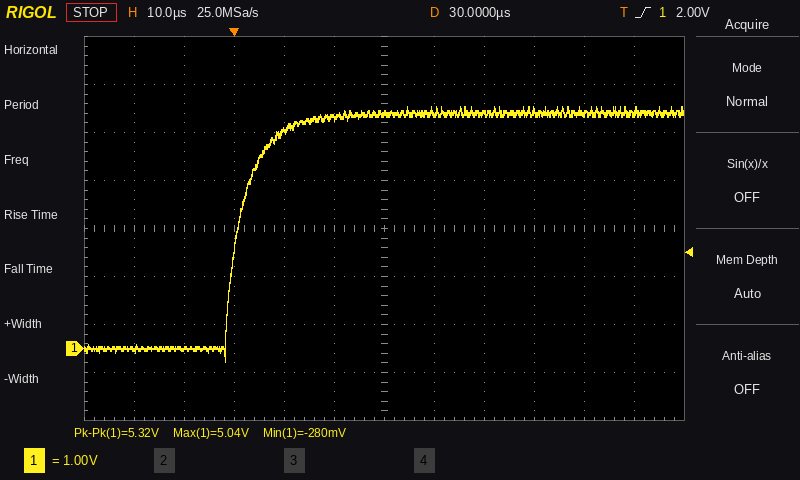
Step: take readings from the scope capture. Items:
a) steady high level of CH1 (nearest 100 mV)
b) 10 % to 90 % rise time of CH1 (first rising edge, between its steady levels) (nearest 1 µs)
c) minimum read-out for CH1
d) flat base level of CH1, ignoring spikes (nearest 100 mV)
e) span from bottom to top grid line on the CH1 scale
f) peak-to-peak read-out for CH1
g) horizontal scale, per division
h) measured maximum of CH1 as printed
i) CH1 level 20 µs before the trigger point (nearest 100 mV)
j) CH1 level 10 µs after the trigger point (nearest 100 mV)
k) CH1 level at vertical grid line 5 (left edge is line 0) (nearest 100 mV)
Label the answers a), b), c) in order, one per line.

a) 4.9 V
b) 10 µs
c) -280 mV
d) 0.0 V
e) 8 V
f) 5.32 V
g) 10 µs
h) 5.04 V
i) 0.0 V
j) 4.5 V
k) 4.8 V
